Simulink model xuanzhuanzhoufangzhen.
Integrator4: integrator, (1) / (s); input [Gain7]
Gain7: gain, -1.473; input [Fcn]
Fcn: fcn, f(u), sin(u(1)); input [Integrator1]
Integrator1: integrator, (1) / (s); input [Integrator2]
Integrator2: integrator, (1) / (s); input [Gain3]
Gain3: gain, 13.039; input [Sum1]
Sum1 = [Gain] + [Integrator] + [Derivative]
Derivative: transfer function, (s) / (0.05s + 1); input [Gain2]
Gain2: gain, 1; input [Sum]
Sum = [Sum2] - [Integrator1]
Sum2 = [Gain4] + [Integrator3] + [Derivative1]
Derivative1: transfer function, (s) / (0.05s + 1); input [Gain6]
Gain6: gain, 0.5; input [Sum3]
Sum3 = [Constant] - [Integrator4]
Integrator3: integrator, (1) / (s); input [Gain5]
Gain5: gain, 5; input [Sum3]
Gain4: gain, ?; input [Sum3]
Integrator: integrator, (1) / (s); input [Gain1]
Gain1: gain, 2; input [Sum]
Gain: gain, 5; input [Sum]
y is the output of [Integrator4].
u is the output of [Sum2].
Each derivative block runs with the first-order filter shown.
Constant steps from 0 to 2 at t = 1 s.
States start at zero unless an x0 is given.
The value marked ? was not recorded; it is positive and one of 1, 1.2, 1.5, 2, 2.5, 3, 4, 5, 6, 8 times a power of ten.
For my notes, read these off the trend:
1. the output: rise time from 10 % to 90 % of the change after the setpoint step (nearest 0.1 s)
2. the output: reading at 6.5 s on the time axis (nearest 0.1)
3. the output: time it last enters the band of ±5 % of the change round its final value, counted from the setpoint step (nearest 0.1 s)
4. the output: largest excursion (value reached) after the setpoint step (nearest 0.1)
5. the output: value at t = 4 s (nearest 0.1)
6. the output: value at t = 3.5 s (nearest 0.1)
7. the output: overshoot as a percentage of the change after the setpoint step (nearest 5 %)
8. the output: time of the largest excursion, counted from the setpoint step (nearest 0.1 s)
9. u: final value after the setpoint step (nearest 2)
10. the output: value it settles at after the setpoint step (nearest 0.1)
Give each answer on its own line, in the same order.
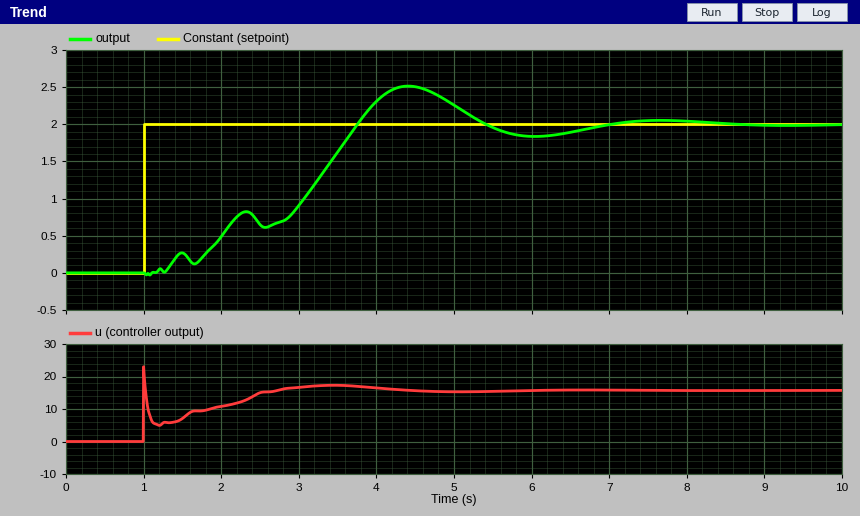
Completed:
2.2 s
1.9
5.5 s
2.5
2.3
1.6
25 %
3.4 s
16
2.0
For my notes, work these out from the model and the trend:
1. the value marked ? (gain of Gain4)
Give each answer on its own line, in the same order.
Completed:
1.5
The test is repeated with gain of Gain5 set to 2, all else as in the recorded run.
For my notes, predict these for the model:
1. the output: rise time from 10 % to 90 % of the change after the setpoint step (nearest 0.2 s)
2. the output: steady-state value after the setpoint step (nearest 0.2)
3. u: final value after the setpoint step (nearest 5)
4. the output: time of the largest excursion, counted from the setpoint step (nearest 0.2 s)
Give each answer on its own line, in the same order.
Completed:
1.2 s
2.0
5
2.8 s
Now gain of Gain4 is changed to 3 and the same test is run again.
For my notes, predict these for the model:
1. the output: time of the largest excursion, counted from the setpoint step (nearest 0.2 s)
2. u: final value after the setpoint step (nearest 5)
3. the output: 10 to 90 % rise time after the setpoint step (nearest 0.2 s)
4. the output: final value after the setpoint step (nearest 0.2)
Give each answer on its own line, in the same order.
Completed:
4.0 s
20
2.0 s
2.0
